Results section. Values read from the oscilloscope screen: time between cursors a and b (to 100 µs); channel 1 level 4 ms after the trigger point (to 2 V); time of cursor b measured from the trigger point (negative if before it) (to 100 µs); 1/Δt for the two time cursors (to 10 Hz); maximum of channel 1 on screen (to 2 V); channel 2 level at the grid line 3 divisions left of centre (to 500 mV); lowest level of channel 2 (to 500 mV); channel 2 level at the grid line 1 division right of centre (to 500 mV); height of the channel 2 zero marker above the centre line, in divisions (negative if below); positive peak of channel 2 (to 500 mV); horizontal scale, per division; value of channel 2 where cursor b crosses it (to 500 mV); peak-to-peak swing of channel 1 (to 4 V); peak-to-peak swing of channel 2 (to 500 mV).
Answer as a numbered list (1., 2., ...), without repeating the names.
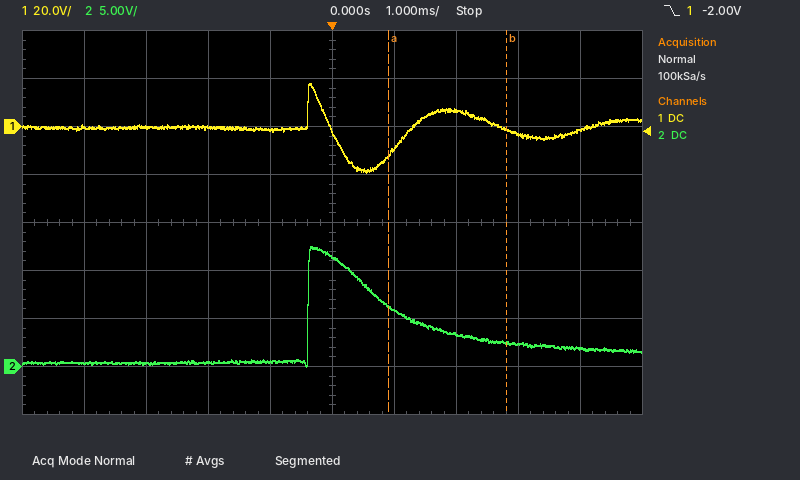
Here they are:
1. 1.9 ms
2. -2 V
3. +2.8 ms
4. 530 Hz
5. 18 V
6. 500 mV
7. 0.0 V
8. 6.0 V
9. -3.0 div
10. 12.5 V
11. 1 ms
12. 2.5 V
13. 36 V
14. 12.5 V
